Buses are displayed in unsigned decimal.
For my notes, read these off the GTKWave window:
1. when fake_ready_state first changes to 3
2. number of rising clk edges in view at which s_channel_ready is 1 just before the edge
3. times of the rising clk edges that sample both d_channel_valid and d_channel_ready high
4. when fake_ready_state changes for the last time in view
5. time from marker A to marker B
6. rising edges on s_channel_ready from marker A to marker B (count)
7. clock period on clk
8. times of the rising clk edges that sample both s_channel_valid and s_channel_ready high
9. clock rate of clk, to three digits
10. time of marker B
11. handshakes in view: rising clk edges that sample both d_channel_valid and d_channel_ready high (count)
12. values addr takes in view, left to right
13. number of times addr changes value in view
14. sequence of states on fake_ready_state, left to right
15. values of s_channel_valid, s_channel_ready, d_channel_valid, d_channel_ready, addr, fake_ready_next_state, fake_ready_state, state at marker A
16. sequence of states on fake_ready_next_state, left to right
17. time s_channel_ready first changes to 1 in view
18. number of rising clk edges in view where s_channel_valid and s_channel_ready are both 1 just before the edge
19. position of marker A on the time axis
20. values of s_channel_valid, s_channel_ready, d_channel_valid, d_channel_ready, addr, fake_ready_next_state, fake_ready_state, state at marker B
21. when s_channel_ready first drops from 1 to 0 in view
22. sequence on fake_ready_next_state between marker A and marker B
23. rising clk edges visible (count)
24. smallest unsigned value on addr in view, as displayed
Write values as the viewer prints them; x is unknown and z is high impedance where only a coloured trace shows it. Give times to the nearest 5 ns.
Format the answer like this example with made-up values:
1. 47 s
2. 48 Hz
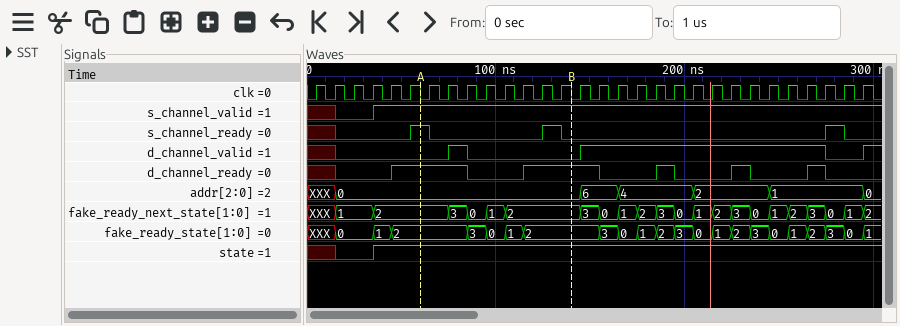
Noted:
1. 85 ns
2. 3
3. 85 ns, 155 ns, 195 ns, 235 ns, 275 ns
4. 295 ns
5. 80 ns
6. 1
7. 10 ns
8. 65 ns, 135 ns, 285 ns
9. 100 MHz
10. 140 ns
11. 5
12. XXX, 0, 6, 4, 2, 1, 0
13. 6
14. XXX, 0, 1, 2, 3, 0, 1, 2, 3, 0, 1, 2, 3, 0, 1, 2, 3, 0, 1, 2, 3, 0, 1
15. s_channel_valid=1, s_channel_ready=1, d_channel_valid=0, d_channel_ready=1, addr=0, fake_ready_next_state=2, fake_ready_state=2, state=1
16. XXX, 1, 2, 3, 0, 1, 2, 3, 0, 1, 2, 3, 0, 1, 2, 3, 0, 1, 2, 3, 0, 1, 2
17. 55 ns
18. 3
19. 60 ns
20. s_channel_valid=1, s_channel_ready=0, d_channel_valid=0, d_channel_ready=1, addr=0, fake_ready_next_state=2, fake_ready_state=2, state=1
21. 65 ns
22. 2, 3, 0, 1, 2
23. 30
24. 0
